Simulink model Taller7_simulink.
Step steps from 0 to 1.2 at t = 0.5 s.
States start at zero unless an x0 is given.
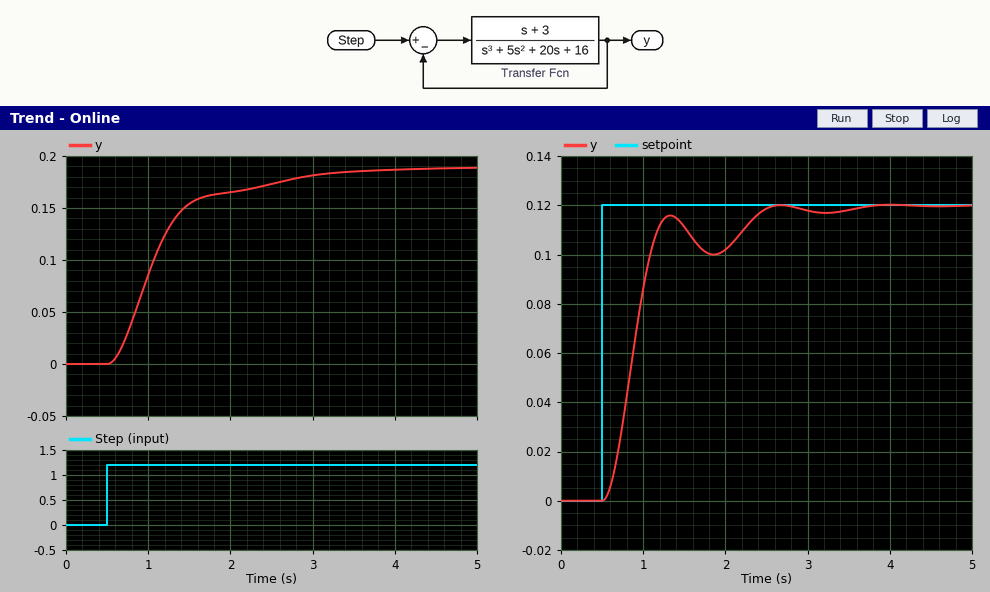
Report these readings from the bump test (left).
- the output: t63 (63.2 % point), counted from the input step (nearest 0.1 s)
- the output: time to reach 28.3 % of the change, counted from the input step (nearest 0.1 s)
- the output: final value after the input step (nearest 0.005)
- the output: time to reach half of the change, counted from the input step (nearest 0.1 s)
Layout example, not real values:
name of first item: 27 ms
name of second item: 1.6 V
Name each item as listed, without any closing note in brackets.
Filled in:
the output: t63 (63.2 % point), counted from the input step: 0.7 s
the output: time to reach 28.3 % of the change, counted from the input step: 0.4 s
the output: final value after the input step: 0.190
the output: time to reach half of the change, counted from the input step: 0.5 s
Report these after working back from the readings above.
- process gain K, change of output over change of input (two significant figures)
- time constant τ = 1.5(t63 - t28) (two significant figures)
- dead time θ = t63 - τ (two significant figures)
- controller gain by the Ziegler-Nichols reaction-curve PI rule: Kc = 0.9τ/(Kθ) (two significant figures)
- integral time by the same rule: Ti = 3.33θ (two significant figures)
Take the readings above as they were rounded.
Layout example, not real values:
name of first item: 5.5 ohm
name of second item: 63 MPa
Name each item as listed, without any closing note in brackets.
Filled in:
process gain K, change of output over change of input: 0.16
time constant τ = 1.5(t63 - t28): 0.45 s
dead time θ = t63 - τ: 0.25 s
controller gain by the Ziegler-Nichols reaction-curve PI rule: Kc = 0.9τ/(Kθ): 10
integral time by the same rule: Ti = 3.33θ: 0.83 s
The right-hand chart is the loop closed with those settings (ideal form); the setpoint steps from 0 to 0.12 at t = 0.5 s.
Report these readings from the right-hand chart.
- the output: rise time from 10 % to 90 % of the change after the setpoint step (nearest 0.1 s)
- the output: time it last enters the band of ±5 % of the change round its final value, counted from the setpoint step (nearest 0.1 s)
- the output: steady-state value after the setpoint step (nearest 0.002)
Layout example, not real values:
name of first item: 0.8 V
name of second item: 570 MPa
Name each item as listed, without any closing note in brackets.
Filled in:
the output: rise time from 10 % to 90 % of the change after the setpoint step: 0.5 s
the output: time it last enters the band of ±5 % of the change round its final value, counted from the setpoint step: 1.8 s
the output: steady-state value after the setpoint step: 0.120
